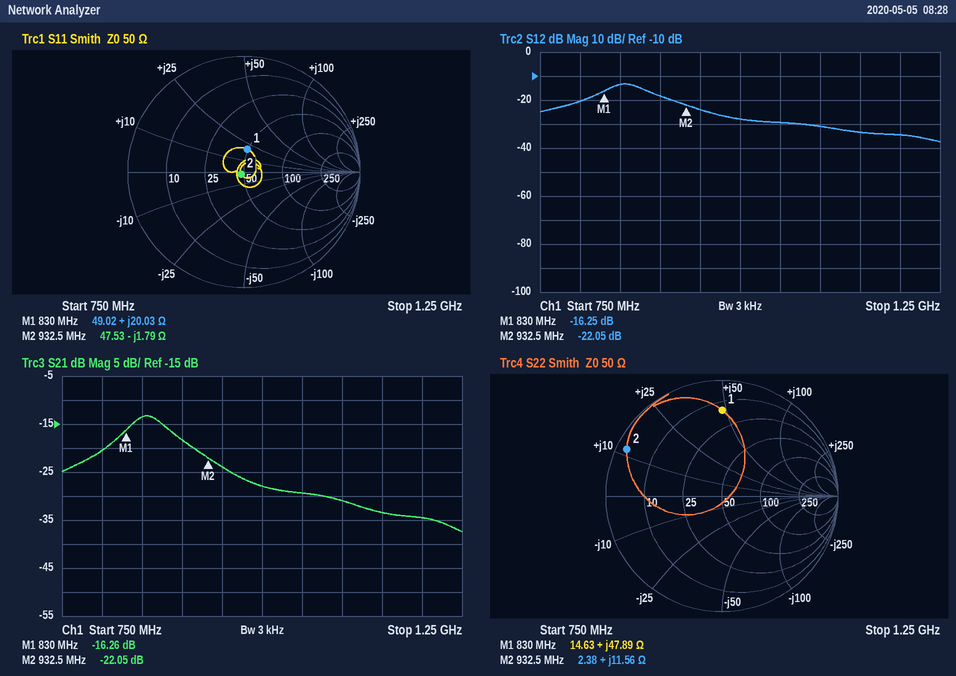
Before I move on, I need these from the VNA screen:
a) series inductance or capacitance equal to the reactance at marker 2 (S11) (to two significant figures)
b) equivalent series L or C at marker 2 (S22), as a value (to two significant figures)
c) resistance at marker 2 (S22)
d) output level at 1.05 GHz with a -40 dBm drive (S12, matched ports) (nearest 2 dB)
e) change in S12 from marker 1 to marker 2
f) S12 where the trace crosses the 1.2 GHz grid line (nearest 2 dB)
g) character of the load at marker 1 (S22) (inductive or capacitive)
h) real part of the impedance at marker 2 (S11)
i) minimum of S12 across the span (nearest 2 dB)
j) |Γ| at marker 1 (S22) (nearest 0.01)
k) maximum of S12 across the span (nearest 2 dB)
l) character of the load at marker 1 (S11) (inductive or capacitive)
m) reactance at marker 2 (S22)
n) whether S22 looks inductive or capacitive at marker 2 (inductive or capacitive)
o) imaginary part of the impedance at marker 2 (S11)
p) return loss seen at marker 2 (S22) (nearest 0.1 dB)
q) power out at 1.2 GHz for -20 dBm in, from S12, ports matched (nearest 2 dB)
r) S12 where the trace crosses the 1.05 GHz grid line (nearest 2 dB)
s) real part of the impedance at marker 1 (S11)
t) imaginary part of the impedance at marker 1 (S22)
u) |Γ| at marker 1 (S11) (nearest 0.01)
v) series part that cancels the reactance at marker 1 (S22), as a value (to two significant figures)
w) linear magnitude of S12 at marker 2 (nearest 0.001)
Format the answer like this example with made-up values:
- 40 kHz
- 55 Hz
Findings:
- 95 pF
- 2.0 nH
- 2.38 Ω
- -70 dBm
- -5.80 dB
- -34 dB
- inductive
- 47.53 Ω
- -38 dB
- 0.74
- -14 dB
- inductive
- +11.56 Ω
- inductive
- -1.79 Ω
- 0.8 dB
- -54 dBm
- -30 dB
- 49.02 Ω
- +47.89 Ω
- 0.20
- 4.0 pF
- 0.079
